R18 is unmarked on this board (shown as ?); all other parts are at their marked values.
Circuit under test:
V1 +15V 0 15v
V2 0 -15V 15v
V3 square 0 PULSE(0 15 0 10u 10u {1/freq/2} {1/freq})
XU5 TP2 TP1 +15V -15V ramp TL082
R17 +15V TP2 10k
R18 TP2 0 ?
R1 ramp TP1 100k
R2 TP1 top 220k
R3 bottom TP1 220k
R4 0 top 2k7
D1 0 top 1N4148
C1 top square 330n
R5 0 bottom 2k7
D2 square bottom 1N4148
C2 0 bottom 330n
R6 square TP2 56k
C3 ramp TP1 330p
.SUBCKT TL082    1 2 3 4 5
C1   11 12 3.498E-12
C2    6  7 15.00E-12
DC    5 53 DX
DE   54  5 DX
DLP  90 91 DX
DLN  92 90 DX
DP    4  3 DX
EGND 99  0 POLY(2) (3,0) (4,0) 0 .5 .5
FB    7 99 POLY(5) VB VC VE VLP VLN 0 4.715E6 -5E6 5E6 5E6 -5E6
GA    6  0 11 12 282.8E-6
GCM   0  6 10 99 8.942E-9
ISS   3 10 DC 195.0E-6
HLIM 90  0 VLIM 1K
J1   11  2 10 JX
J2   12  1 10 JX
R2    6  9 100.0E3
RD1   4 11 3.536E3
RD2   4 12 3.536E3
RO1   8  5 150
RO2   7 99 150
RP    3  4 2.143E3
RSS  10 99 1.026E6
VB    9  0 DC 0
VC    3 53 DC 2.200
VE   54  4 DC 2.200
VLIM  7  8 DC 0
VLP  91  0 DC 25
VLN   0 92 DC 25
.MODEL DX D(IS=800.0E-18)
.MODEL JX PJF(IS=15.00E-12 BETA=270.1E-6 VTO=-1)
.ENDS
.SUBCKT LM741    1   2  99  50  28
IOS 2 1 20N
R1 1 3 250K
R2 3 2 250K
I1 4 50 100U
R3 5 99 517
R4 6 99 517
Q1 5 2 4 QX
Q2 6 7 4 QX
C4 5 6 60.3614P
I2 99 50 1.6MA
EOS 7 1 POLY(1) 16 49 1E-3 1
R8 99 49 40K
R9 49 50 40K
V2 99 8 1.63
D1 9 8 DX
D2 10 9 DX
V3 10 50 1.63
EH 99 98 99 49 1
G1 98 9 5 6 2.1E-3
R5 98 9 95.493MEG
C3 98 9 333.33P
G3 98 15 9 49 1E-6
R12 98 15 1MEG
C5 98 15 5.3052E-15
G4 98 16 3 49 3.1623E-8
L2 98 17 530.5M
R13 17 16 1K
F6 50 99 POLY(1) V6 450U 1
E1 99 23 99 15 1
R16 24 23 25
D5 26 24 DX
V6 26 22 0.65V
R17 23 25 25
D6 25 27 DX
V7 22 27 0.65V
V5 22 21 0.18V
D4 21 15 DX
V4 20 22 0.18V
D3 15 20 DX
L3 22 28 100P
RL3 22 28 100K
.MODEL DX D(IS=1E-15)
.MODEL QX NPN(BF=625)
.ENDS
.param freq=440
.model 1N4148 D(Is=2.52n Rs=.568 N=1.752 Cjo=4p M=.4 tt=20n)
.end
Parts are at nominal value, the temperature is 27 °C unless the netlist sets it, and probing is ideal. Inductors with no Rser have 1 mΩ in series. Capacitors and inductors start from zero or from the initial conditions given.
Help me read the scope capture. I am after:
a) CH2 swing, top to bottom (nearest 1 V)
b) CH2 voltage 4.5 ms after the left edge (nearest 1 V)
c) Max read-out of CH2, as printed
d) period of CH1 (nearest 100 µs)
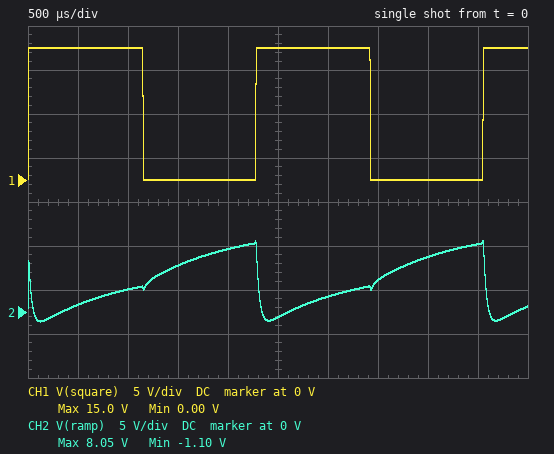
9 V
8 V
8.05 V
2.3 ms
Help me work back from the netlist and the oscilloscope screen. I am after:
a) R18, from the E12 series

5.6 kΩ
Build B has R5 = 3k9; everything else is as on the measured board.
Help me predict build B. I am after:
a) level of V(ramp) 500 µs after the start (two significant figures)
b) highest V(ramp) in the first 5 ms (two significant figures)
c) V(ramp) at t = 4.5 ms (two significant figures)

810 mV
7.2 V
6.8 V
